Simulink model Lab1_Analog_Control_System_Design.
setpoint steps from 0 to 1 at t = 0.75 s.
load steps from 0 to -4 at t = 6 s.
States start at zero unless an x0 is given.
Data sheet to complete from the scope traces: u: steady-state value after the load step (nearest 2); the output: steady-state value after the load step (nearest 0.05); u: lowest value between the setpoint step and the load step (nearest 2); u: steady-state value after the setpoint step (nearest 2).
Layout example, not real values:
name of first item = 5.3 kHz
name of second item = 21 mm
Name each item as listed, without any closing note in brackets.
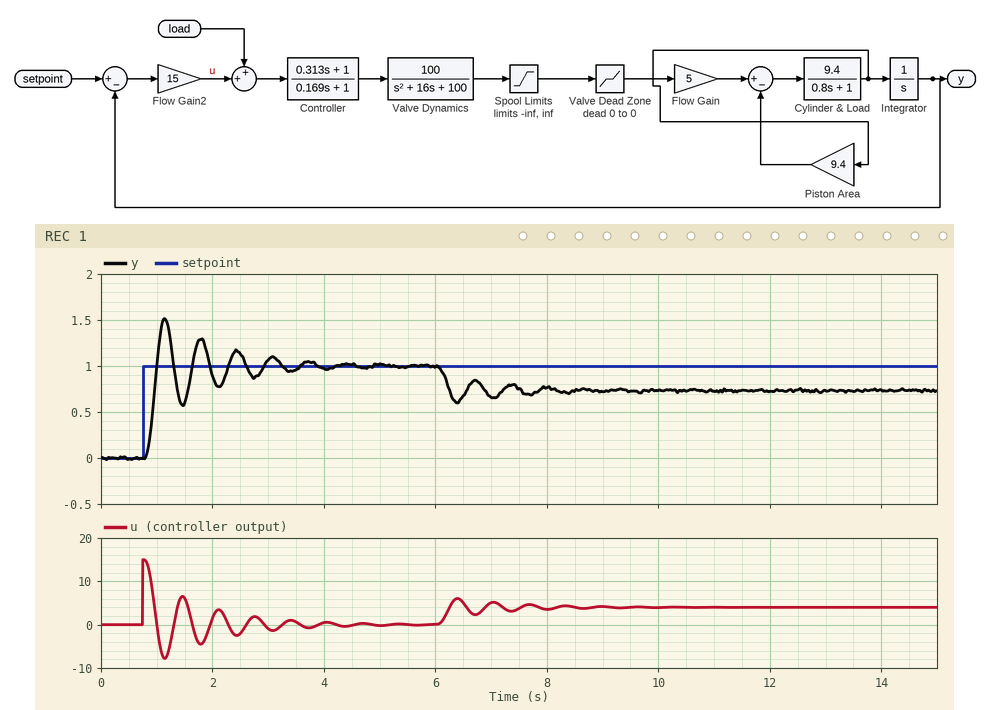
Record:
u: steady-state value after the load step = 4
the output: steady-state value after the load step = 0.75
u: lowest value between the setpoint step and the load step = -8
u: steady-state value after the setpoint step = 0
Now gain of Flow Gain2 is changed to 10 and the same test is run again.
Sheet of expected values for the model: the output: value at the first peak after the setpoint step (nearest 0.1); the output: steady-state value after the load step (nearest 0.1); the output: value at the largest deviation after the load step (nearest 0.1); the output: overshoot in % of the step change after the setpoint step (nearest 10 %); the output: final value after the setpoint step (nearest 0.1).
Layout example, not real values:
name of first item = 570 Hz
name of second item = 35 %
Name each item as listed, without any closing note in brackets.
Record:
the output: value at the first peak after the setpoint step = 1.3
the output: steady-state value after the load step = 0.6
the output: value at the largest deviation after the load step = 0.5
the output: overshoot in % of the step change after the setpoint step = 30 %
the output: final value after the setpoint step = 1.0
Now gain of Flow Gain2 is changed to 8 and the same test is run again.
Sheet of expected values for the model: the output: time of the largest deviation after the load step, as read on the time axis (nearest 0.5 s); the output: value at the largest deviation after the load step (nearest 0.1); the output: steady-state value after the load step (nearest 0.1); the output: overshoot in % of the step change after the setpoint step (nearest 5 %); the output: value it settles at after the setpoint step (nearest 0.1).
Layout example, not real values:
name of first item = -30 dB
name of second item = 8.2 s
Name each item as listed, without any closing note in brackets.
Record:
the output: time of the largest deviation after the load step, as read on the time axis = 6.5 s
the output: value at the largest deviation after the load step = 0.4
the output: steady-state value after the load step = 0.5
the output: overshoot in % of the step change after the setpoint step = 15 %
the output: value it settles at after the setpoint step = 1.0
